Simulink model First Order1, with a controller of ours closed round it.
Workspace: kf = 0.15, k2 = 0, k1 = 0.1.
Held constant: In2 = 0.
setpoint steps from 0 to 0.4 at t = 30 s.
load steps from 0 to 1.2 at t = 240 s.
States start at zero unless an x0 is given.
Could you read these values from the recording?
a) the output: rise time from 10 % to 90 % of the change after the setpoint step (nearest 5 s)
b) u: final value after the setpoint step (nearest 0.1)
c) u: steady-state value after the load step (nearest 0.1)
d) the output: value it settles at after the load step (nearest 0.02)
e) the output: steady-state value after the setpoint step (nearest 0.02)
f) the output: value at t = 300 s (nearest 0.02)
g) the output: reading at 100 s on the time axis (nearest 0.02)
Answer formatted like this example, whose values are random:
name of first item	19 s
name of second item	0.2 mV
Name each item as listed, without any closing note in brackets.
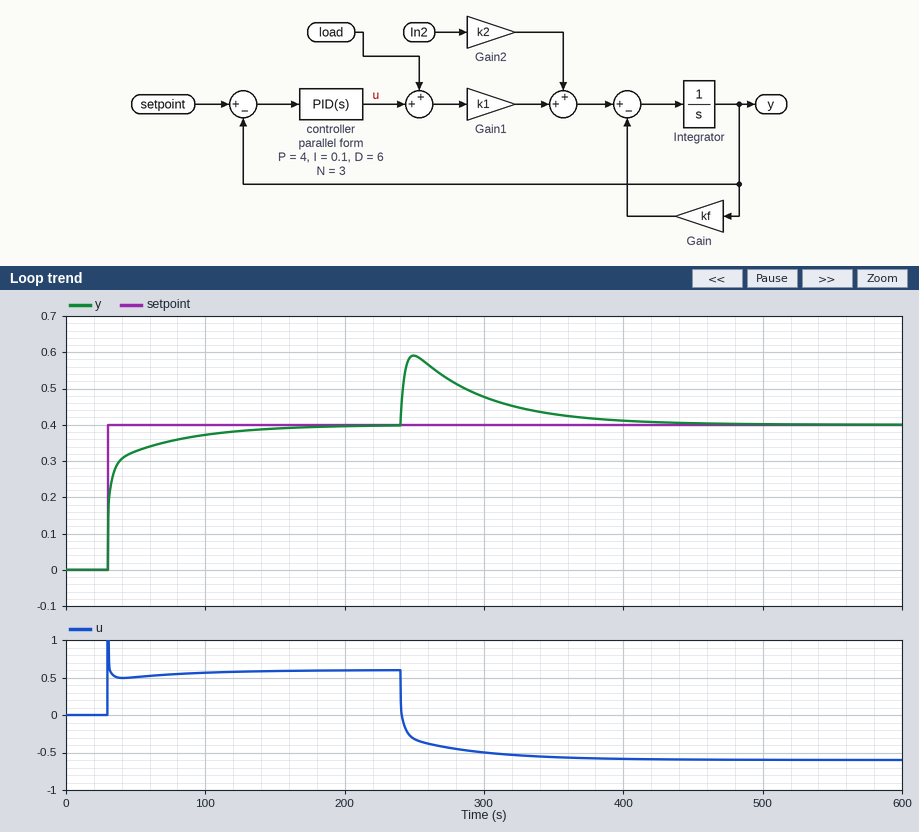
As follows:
the output: rise time from 10 % to 90 % of the change after the setpoint step	50 s
u: final value after the setpoint step	0.6
u: steady-state value after the load step	-0.6
the output: value it settles at after the load step	0.40
the output: steady-state value after the setpoint step	0.40
the output: value at t = 300 s	0.48
the output: reading at 100 s on the time axis	0.38
